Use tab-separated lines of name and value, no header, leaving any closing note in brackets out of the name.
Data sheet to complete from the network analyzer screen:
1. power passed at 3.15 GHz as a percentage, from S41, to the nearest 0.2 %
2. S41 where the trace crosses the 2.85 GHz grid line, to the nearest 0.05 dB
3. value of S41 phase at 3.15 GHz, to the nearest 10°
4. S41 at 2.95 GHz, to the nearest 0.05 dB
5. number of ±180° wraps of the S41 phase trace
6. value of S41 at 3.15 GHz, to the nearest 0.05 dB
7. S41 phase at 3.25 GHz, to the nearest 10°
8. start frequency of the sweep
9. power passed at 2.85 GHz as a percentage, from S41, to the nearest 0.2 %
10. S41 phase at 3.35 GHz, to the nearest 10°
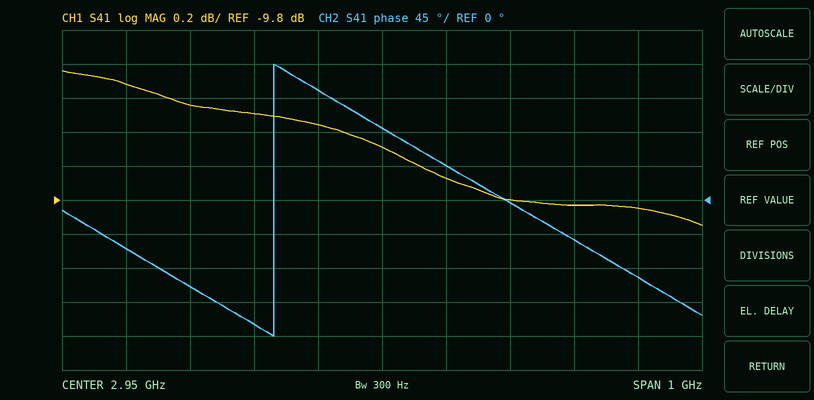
power passed at 3.15 GHz as a percentage, from S41, to the nearest 0.2 %	10.4 %
S41 where the trace crosses the 2.85 GHz grid line, to the nearest 0.05 dB	-9.35 dB
value of S41 phase at 3.15 GHz, to the nearest 10°	0°
S41 at 2.95 GHz, to the nearest 0.05 dB	-9.50 dB
number of ±180° wraps of the S41 phase trace	1
value of S41 at 3.15 GHz, to the nearest 0.05 dB	-9.80 dB
S41 phase at 3.25 GHz, to the nearest 10°	-50°
start frequency of the sweep	2.45 GHz
power passed at 2.85 GHz as a percentage, from S41, to the nearest 0.2 %	11.6 %
S41 phase at 3.35 GHz, to the nearest 10°	-100°
